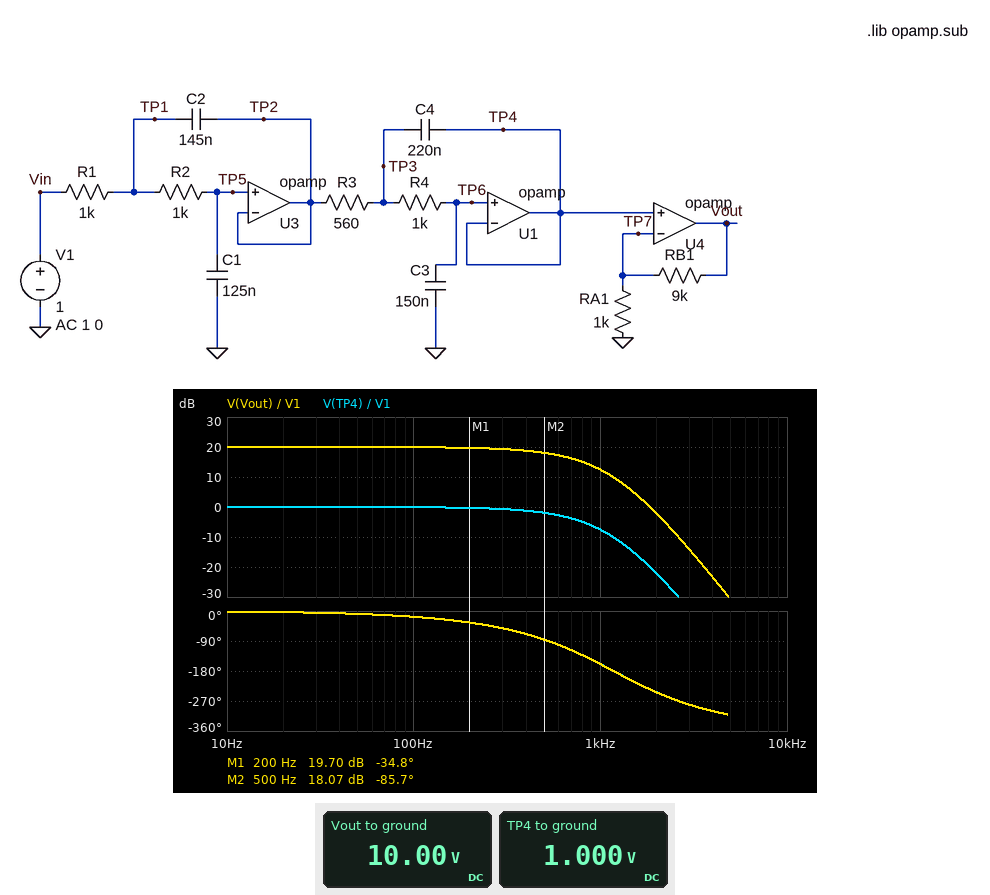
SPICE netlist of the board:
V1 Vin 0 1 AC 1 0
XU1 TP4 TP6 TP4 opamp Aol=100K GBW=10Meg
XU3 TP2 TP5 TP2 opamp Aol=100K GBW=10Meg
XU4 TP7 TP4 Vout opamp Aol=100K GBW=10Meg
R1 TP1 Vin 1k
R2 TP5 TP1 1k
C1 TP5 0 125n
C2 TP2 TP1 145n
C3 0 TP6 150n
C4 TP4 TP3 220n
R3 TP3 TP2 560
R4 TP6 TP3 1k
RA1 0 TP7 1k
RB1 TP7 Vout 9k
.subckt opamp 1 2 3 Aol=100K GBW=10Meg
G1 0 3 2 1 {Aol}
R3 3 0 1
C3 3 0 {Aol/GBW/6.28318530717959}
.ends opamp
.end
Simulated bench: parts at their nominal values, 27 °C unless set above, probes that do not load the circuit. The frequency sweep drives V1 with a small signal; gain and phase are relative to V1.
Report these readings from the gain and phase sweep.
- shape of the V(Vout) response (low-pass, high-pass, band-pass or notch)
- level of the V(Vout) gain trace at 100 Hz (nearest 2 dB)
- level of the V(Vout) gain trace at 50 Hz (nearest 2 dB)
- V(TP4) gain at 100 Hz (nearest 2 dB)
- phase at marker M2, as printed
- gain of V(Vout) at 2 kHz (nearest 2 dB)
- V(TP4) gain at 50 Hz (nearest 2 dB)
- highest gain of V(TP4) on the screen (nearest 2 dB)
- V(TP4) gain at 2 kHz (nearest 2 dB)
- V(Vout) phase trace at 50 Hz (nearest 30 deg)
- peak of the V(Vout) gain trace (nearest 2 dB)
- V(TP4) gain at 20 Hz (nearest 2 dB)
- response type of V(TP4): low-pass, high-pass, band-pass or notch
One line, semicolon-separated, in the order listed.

low-pass; 20 dB; 20 dB; 0 dB; -85.7 deg; -2 dB; 0 dB; 0 dB; -22 dB; 0 deg; 20 dB; 0 dB; low-pass
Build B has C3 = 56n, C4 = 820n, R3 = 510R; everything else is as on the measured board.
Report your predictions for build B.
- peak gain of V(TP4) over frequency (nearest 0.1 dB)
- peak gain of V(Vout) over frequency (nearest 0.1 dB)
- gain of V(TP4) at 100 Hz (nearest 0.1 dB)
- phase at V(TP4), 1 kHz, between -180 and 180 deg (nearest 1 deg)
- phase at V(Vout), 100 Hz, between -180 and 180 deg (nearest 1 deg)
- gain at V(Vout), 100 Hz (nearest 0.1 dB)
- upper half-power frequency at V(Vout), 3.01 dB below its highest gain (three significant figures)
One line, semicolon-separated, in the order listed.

2.0 dB; 22.0 dB; 0 dB; -162 deg; -12 deg; 20.0 dB; 1.13 kHz
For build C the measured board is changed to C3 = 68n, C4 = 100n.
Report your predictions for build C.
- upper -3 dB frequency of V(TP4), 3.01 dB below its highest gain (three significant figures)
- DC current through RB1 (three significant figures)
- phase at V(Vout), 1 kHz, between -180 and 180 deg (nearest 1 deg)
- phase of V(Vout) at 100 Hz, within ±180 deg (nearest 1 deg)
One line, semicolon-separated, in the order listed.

782 Hz; 1.00 mA; -118 deg; -13 deg
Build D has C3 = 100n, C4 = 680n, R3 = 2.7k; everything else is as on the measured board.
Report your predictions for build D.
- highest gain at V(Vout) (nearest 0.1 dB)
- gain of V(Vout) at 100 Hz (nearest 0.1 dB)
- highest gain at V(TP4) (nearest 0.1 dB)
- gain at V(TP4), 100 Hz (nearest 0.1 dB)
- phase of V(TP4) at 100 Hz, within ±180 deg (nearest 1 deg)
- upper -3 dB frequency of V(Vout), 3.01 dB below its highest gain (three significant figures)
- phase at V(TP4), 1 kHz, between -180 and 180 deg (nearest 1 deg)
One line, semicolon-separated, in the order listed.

21.8 dB; 20.3 dB; 1.8 dB; 0.3 dB; -23 deg; 428 Hz; 121 deg
